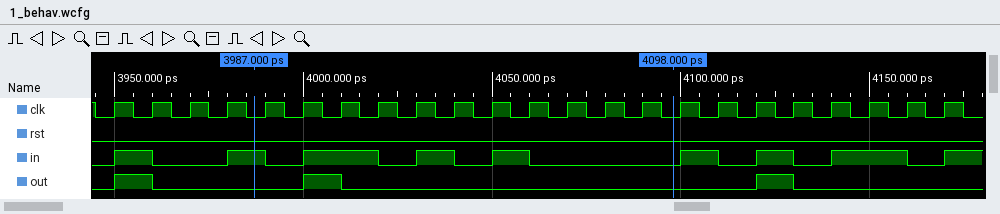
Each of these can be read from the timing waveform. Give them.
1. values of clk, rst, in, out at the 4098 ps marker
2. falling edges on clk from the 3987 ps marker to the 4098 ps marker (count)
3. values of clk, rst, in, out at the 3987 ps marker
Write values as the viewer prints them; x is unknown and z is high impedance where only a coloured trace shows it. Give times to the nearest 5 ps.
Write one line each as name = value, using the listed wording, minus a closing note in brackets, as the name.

values of clk, rst, in, out at the 4098 ps marker = clk=0, rst=0, in=0, out=0
falling edges on clk from the 3987 ps marker to the 4098 ps marker = 11
values of clk, rst, in, out at the 3987 ps marker = clk=0, rst=0, in=1, out=0
